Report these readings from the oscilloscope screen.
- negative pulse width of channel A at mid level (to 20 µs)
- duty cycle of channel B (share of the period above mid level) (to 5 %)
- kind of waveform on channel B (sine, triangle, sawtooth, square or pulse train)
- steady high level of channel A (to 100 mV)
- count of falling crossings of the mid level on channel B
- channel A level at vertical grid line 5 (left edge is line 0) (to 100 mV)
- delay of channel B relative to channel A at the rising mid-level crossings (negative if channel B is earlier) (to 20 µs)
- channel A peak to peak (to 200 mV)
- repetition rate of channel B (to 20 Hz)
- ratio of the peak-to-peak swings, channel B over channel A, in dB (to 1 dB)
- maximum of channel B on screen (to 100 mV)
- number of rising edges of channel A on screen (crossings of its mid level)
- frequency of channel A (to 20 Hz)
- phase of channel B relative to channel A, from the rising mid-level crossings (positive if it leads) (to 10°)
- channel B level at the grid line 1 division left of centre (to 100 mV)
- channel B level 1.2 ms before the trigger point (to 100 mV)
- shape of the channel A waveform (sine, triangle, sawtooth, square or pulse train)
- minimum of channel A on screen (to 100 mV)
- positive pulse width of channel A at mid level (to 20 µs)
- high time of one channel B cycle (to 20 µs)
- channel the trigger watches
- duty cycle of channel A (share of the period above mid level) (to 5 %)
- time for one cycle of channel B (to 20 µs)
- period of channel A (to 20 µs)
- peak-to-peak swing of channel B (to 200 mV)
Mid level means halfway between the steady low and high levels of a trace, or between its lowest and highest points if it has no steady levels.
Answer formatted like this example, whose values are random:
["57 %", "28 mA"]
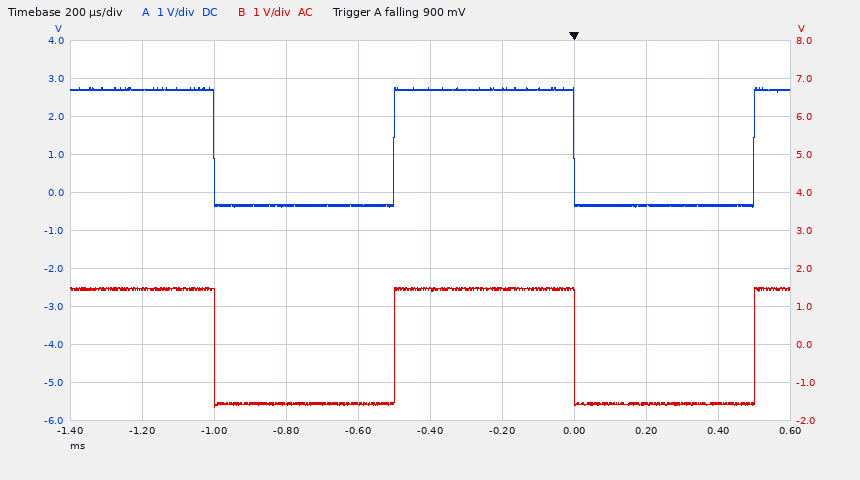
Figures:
["500 µs", "50 %", "square", "2.7 V", "2", "2.7 V", "0 µs", "3.2 V", "1.00 kHz", "0 dB", "1.5 V", "2", "1.00 kHz", "0°", "-1.6 V", "1.5 V", "square", "-400 mV", "500 µs", "500 µs", "channel A", "50 %", "1.00 ms", "1.00 ms", "3.2 V"]
